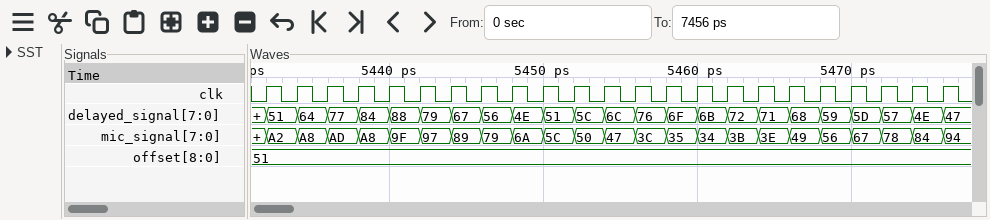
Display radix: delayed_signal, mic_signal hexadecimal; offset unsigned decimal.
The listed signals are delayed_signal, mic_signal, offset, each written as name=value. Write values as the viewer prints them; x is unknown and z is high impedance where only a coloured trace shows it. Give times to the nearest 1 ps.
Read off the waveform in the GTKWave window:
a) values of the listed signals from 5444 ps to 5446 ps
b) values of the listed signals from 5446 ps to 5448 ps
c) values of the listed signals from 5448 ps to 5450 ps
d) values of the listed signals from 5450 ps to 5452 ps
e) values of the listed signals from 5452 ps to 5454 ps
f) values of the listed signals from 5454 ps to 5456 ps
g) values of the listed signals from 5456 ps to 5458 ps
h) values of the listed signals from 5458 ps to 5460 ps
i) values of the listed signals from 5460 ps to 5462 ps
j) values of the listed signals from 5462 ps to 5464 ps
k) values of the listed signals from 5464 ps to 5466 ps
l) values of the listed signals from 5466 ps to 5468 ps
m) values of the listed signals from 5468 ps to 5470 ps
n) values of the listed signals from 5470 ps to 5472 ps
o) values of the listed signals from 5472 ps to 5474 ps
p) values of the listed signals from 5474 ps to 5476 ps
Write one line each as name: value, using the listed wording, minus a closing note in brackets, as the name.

values of the listed signals from 5444 ps to 5446 ps: delayed_signal=67, mic_signal=89, offset=51
values of the listed signals from 5446 ps to 5448 ps: delayed_signal=56, mic_signal=79, offset=51
values of the listed signals from 5448 ps to 5450 ps: delayed_signal=4E, mic_signal=6A, offset=51
values of the listed signals from 5450 ps to 5452 ps: delayed_signal=51, mic_signal=5C, offset=51
values of the listed signals from 5452 ps to 5454 ps: delayed_signal=5C, mic_signal=50, offset=51
values of the listed signals from 5454 ps to 5456 ps: delayed_signal=6C, mic_signal=47, offset=51
values of the listed signals from 5456 ps to 5458 ps: delayed_signal=76, mic_signal=3C, offset=51
values of the listed signals from 5458 ps to 5460 ps: delayed_signal=6F, mic_signal=35, offset=51
values of the listed signals from 5460 ps to 5462 ps: delayed_signal=6B, mic_signal=34, offset=51
values of the listed signals from 5462 ps to 5464 ps: delayed_signal=72, mic_signal=3B, offset=51
values of the listed signals from 5464 ps to 5466 ps: delayed_signal=71, mic_signal=3E, offset=51
values of the listed signals from 5466 ps to 5468 ps: delayed_signal=68, mic_signal=49, offset=51
values of the listed signals from 5468 ps to 5470 ps: delayed_signal=59, mic_signal=56, offset=51
values of the listed signals from 5470 ps to 5472 ps: delayed_signal=5D, mic_signal=67, offset=51
values of the listed signals from 5472 ps to 5474 ps: delayed_signal=57, mic_signal=78, offset=51
values of the listed signals from 5474 ps to 5476 ps: delayed_signal=4E, mic_signal=84, offset=51
